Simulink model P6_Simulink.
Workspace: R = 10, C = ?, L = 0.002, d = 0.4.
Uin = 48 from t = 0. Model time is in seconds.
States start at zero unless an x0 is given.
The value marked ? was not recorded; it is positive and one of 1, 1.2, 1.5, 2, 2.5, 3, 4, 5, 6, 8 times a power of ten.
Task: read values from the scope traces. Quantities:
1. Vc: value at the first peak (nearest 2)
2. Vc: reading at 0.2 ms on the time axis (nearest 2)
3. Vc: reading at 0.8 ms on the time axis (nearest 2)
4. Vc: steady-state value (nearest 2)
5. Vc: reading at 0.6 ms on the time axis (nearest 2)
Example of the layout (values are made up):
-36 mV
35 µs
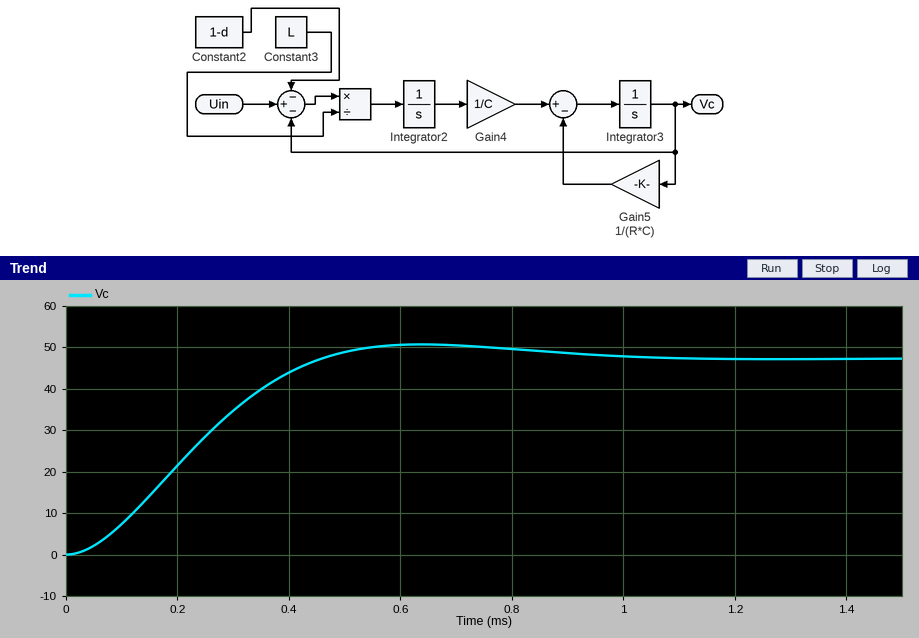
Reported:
50
22
50
48
50
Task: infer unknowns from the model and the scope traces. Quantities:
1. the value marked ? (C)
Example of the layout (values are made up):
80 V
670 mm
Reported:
1.2e-05
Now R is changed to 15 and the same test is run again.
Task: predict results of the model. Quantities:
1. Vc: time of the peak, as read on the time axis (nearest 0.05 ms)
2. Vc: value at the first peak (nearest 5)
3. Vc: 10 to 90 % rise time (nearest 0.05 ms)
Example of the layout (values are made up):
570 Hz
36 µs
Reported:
0.55 ms
60
0.25 ms
